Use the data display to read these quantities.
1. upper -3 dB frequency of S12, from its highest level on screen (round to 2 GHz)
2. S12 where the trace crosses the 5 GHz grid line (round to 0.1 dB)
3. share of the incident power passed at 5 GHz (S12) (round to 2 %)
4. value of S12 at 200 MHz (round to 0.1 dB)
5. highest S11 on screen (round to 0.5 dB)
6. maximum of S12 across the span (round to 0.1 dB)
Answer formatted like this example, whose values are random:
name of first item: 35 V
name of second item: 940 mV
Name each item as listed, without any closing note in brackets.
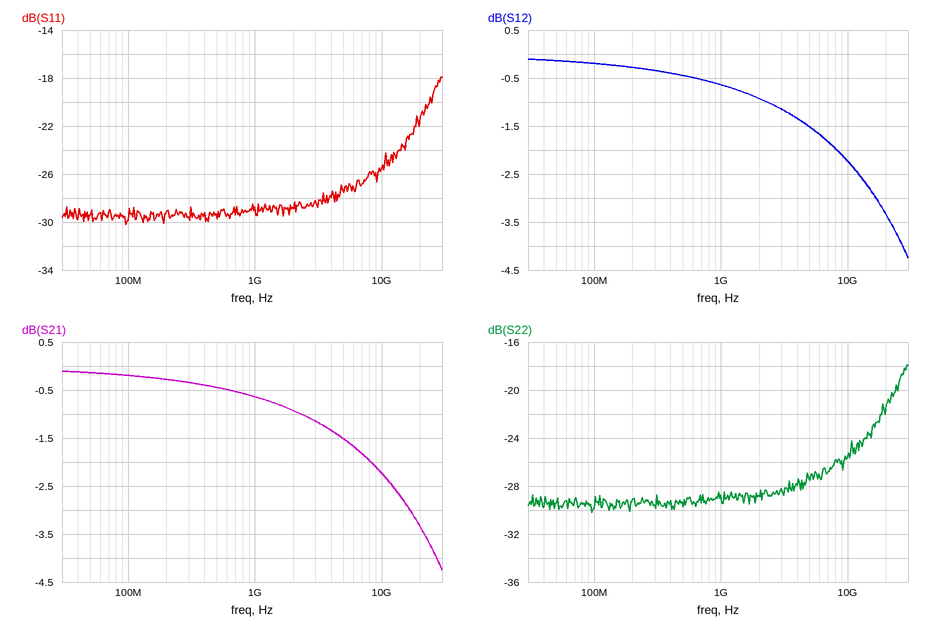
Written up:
upper -3 dB frequency of S12, from its highest level on screen: 18 GHz
S12 where the trace crosses the 5 GHz grid line: -1.5 dB
share of the incident power passed at 5 GHz (S12): 70 %
value of S12 at 200 MHz: -0.3 dB
highest S11 on screen: -18.0 dB
maximum of S12 across the span: -0.1 dB
